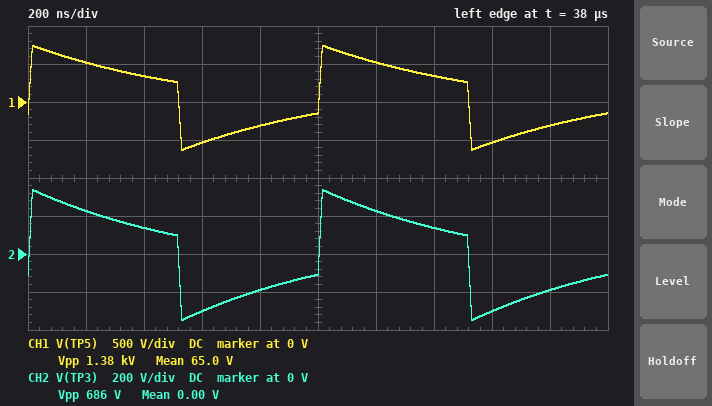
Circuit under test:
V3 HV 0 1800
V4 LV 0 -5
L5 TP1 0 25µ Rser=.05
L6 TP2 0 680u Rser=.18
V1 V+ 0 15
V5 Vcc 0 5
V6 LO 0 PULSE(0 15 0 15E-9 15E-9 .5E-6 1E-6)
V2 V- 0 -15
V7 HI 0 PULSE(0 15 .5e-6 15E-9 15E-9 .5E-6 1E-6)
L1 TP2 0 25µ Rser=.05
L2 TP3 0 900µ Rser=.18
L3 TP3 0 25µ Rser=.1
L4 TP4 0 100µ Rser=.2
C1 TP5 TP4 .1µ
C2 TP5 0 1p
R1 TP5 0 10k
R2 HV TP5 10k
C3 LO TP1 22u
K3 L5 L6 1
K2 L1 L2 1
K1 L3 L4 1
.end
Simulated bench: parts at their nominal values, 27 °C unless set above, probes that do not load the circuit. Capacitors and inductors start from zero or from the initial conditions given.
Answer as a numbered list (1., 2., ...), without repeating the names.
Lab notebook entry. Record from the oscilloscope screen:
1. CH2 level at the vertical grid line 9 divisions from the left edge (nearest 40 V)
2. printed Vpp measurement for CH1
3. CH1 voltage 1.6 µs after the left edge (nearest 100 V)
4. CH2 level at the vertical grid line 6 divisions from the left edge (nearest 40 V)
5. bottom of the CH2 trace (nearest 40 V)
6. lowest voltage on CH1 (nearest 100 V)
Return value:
1. -200 V
2. 1.38 kV
3. -500 V
4. 240 V
5. -360 V
6. -600 V
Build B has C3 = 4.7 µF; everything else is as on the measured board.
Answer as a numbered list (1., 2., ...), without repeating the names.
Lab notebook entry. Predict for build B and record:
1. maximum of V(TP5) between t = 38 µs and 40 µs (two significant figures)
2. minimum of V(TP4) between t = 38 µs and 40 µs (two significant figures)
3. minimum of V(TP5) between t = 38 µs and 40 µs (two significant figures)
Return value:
1. 830 V
2. -790 V
3. -720 V
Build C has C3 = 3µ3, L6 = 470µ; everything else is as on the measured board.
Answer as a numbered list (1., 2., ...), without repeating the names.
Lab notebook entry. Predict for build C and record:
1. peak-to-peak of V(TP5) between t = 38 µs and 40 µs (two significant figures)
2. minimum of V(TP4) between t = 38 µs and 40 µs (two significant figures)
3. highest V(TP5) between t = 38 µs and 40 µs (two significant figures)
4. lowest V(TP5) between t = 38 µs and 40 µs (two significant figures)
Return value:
1. 1.2 kV
2. -620 V
3. 660 V
4. -550 V
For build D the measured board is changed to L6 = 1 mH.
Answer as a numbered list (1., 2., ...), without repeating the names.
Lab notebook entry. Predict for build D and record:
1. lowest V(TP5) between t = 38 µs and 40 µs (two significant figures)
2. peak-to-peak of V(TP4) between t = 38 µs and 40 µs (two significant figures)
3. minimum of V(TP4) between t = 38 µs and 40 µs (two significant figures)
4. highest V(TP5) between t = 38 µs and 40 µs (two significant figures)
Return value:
1. -840 V
2. 1.8 kV
3. -910 V
4. 950 V
